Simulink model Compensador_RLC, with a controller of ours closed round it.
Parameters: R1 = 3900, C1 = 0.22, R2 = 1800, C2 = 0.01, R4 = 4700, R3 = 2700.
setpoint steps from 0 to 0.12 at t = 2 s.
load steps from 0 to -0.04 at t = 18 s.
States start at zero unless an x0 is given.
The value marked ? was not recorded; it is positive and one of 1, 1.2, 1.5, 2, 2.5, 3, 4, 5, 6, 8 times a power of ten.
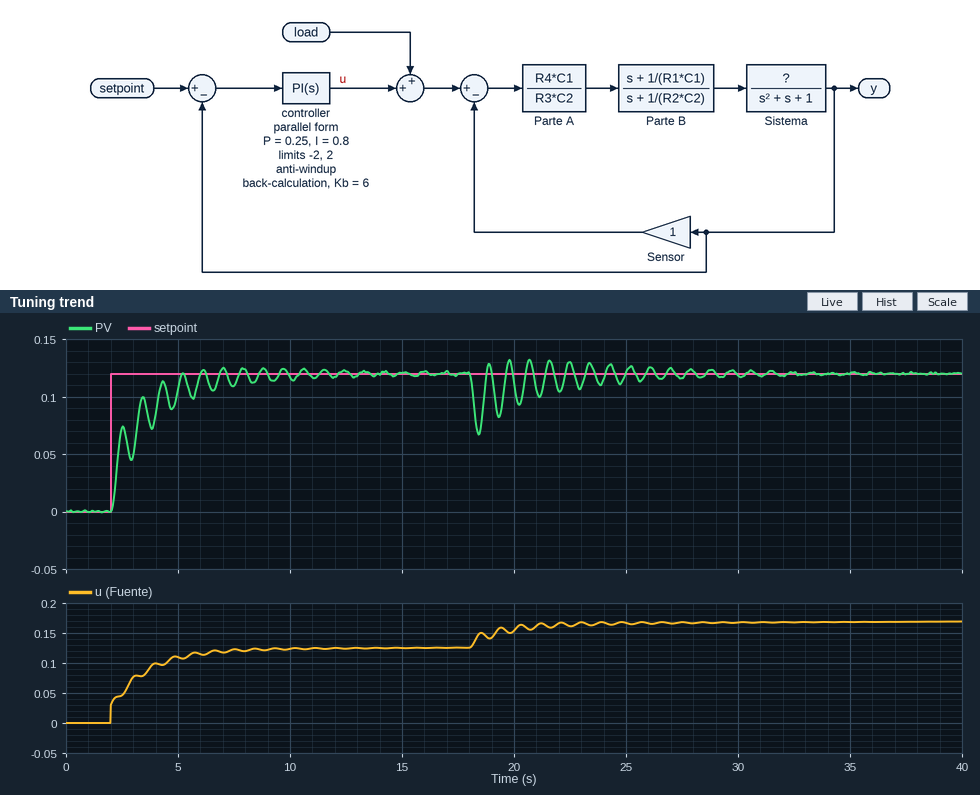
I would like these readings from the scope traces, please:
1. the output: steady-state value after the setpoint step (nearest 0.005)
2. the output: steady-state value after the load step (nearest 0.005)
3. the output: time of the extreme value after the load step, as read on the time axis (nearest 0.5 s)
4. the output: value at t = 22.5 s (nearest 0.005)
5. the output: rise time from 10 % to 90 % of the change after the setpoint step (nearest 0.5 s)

0.120
0.120
18.5 s
0.130
2.0 s
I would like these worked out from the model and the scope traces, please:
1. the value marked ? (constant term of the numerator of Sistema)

1
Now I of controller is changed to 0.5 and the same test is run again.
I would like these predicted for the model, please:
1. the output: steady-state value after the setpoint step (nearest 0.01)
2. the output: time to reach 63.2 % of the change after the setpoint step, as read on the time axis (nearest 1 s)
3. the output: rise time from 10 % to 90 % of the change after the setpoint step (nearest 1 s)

0.12
3 s
5 s
